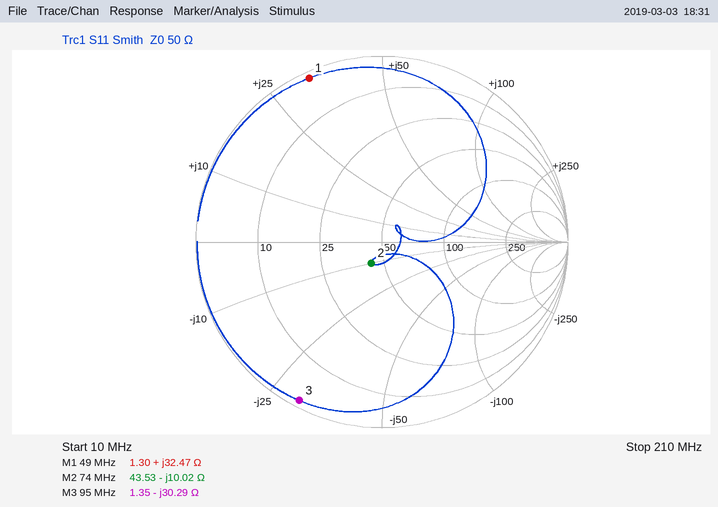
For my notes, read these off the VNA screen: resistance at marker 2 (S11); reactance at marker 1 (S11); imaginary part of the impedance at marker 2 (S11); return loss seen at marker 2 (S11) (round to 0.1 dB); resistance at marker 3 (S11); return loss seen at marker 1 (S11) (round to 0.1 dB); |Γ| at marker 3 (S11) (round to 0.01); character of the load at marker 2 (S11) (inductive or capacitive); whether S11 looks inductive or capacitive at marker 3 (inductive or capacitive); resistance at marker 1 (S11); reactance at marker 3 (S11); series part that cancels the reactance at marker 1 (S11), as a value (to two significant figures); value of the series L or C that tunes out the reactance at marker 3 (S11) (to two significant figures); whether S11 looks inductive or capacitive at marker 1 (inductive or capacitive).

43.53 Ω
+32.47 Ω
-10.02 Ω
17.9 dB
1.35 Ω
0.3 dB
0.96
capacitive
capacitive
1.30 Ω
-30.29 Ω
100 pF
51 nH
inductive
